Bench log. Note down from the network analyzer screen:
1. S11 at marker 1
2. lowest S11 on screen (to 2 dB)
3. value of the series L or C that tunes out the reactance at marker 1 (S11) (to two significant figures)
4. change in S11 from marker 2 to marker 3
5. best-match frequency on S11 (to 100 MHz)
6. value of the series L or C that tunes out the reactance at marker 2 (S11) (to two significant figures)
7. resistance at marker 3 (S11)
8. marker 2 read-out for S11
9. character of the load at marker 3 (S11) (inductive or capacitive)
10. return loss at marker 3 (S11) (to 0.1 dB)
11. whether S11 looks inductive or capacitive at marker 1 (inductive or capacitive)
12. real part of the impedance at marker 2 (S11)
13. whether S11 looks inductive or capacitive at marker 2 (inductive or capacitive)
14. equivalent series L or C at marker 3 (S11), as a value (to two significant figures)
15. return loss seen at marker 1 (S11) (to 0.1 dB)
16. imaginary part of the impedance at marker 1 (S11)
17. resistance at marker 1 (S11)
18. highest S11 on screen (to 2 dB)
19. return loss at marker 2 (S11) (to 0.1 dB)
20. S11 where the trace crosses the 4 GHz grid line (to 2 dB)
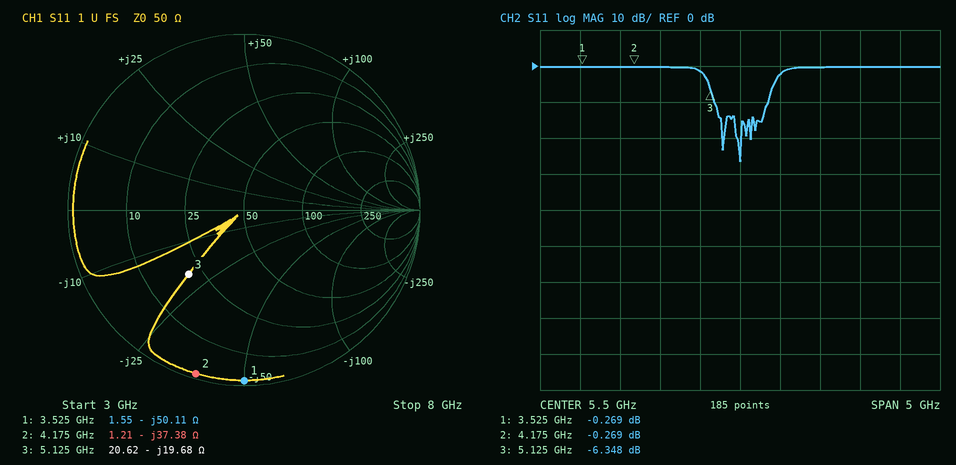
-0.269 dB
-26 dB
2.3 nH
-6.079 dB
5.5 GHz
1.4 nH
20.62 Ω
-0.269 dB
capacitive
6.3 dB
capacitive
1.21 Ω
capacitive
1.6 pF
0.3 dB
-50.11 Ω
1.55 Ω
0 dB
0.3 dB
0 dB
